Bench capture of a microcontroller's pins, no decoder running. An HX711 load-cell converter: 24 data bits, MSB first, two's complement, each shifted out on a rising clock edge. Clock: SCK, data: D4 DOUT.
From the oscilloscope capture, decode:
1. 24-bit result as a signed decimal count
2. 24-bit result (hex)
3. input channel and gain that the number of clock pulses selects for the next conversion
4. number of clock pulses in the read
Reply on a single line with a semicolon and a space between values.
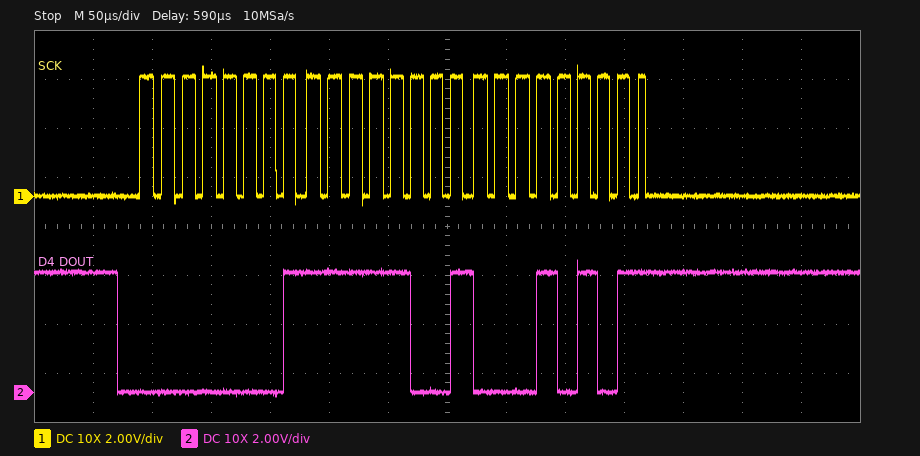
129301; 0x01F915; channel A, gain 128; 25
